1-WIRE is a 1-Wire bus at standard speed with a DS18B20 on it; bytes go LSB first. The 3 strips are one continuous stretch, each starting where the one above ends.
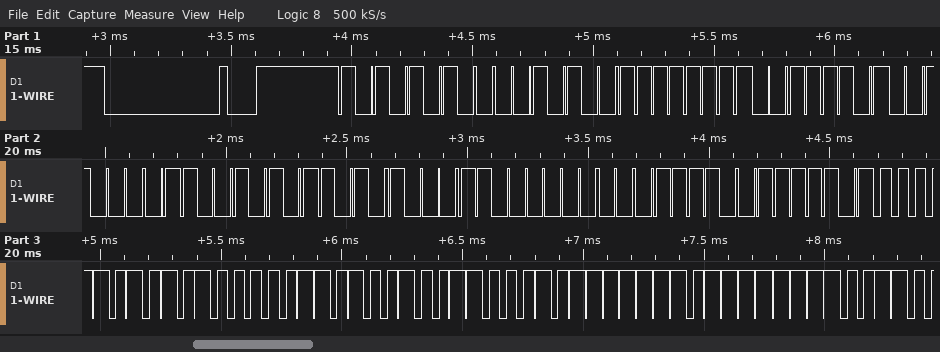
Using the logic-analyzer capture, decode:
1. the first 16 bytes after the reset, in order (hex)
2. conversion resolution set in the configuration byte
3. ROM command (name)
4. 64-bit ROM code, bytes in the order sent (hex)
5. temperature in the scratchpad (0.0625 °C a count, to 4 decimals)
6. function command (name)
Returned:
55 28 FF BC 84 A9 15 03 78 BE 50 05 4B 46 7F FF
12 bits
Match ROM
28 FF BC 84 A9 15 03 78
85.0000 °C
Read Scratchpad
